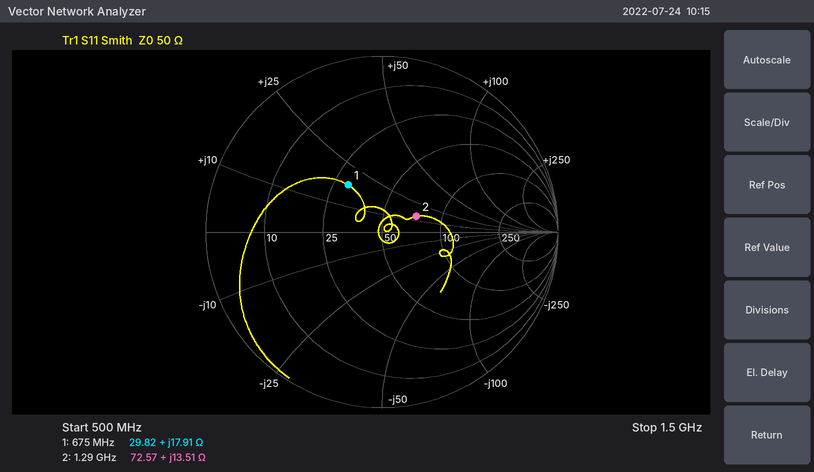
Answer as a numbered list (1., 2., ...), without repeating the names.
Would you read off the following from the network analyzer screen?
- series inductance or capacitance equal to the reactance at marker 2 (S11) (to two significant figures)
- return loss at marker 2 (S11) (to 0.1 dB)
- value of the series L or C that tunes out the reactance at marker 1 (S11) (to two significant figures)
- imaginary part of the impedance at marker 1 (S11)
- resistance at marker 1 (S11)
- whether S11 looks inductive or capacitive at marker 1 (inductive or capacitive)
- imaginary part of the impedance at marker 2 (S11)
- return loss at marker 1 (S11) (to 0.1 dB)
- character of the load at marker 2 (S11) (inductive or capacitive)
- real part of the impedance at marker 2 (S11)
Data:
1. 1.7 nH
2. 13.4 dB
3. 13 pF
4. +17.91 Ω
5. 29.82 Ω
6. inductive
7. +13.51 Ω
8. 9.6 dB
9. inductive
10. 72.57 Ω
